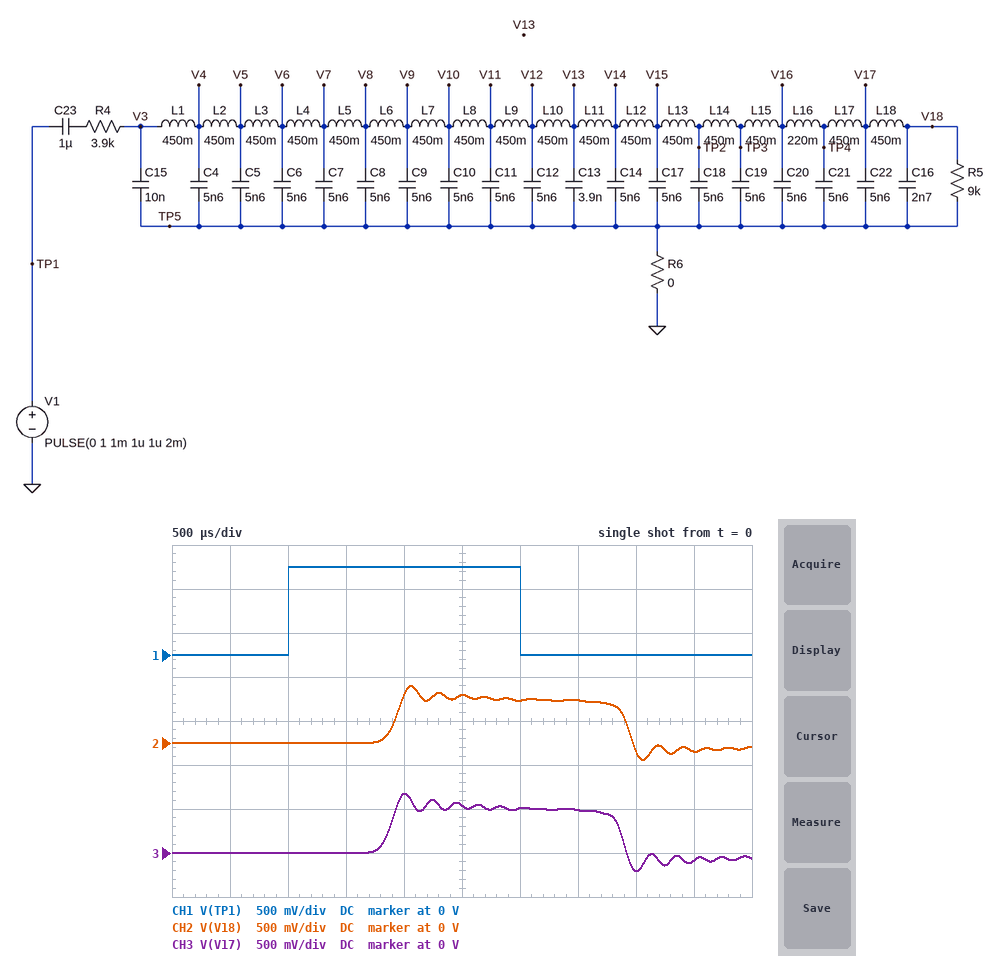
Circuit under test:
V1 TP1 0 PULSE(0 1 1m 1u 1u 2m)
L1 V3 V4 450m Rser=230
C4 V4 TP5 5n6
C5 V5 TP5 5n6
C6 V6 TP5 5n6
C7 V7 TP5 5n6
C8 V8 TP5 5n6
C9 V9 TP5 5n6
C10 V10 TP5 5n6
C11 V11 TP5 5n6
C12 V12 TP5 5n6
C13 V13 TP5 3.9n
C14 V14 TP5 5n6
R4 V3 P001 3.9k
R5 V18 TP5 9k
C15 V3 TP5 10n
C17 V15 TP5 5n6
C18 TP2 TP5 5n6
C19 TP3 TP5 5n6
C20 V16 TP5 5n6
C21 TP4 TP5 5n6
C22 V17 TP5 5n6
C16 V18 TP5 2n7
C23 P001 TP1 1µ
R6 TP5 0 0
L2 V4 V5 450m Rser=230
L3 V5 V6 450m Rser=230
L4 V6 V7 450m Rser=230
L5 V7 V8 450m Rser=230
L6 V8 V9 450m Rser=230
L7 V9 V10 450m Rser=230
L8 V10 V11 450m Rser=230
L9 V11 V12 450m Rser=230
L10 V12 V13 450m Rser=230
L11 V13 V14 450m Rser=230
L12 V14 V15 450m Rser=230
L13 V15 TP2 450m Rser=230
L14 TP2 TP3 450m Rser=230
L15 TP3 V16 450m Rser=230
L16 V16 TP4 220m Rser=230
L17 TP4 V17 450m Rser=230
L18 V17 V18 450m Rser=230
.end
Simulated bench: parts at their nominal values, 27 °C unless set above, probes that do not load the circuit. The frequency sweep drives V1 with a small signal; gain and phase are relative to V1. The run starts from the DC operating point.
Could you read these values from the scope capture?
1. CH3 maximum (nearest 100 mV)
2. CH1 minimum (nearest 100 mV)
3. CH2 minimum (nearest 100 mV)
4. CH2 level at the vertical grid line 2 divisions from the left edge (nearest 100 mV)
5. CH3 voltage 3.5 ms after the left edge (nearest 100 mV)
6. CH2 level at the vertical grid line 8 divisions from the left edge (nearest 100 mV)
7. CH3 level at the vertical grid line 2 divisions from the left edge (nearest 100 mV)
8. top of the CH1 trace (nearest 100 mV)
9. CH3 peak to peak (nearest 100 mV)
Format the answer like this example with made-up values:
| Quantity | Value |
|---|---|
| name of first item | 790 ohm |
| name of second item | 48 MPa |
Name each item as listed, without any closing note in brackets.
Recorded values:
| Quantity | Value |
|---|---|
| CH3 maximum | 700 mV |
| CH1 minimum | 0 V |
| CH2 minimum | -200 mV |
| CH2 level at the vertical grid line 2 divisions from the left edge | 0 V |
| CH3 voltage 3.5 ms after the left edge | 500 mV |
| CH2 level at the vertical grid line 8 divisions from the left edge | -100 mV |
| CH3 level at the vertical grid line 2 divisions from the left edge | 0 V |
| top of the CH1 trace | 1.0 V |
| CH3 peak to peak | 900 mV |
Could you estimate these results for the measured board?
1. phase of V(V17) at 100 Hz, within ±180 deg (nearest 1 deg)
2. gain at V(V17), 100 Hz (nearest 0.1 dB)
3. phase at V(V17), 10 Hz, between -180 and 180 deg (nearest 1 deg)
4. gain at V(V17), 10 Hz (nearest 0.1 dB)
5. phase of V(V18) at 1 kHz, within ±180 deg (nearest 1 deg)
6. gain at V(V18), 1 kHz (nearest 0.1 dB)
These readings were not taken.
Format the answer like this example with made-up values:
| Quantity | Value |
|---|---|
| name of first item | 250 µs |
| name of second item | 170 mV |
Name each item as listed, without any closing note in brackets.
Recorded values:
| Quantity | Value |
|---|---|
| phase of V(V17) at 100 Hz, within ±180 deg | -24 deg |
| gain at V(V17), 100 Hz | -5.4 dB |
| phase at V(V17), 10 Hz, between -180 and 180 deg | 40 deg |
| gain at V(V17), 10 Hz | -8.1 dB |
| phase of V(V18) at 1 kHz, within ±180 deg | 33 deg |
| gain at V(V18), 1 kHz | -5.3 dB |
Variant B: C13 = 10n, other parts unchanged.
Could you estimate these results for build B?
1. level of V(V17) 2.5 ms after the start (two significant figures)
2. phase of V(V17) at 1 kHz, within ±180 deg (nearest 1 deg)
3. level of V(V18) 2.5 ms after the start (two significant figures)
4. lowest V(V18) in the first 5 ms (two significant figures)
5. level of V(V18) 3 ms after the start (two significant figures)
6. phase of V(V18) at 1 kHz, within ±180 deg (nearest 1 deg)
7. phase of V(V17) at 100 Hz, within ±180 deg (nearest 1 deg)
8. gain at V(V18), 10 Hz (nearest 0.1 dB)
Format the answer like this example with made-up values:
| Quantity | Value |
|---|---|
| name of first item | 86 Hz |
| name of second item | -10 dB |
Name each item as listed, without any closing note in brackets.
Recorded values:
| Quantity | Value |
|---|---|
| level of V(V17) 2.5 ms after the start | 560 mV |
| phase of V(V17) at 1 kHz, within ±180 deg | 44 deg |
| level of V(V18) 2.5 ms after the start | 520 mV |
| lowest V(V18) in the first 5 ms | -180 mV |
| level of V(V18) 3 ms after the start | 510 mV |
| phase of V(V18) at 1 kHz, within ±180 deg | 26 deg |
| phase of V(V17) at 100 Hz, within ±180 deg | -25 deg |
| gain at V(V18), 10 Hz | -8.4 dB |
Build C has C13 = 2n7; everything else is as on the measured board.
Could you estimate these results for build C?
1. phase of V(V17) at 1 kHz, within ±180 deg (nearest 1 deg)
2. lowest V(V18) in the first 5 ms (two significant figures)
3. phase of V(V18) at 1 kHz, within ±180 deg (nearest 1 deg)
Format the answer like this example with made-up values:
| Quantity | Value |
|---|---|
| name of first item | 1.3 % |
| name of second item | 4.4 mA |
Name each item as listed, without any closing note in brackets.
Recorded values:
| Quantity | Value |
|---|---|
| phase of V(V17) at 1 kHz, within ±180 deg | 52 deg |
| lowest V(V18) in the first 5 ms | -180 mV |
| phase of V(V18) at 1 kHz, within ±180 deg | 34 deg |
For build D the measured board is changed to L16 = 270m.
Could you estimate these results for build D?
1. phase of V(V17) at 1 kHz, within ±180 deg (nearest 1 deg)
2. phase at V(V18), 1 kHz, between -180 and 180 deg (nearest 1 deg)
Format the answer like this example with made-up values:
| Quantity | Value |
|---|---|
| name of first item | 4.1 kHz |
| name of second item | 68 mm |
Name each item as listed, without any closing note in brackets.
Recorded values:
| Quantity | Value |
|---|---|
| phase of V(V17) at 1 kHz, within ±180 deg | 50 deg |
| phase at V(V18), 1 kHz, between -180 and 180 deg | 32 deg |
